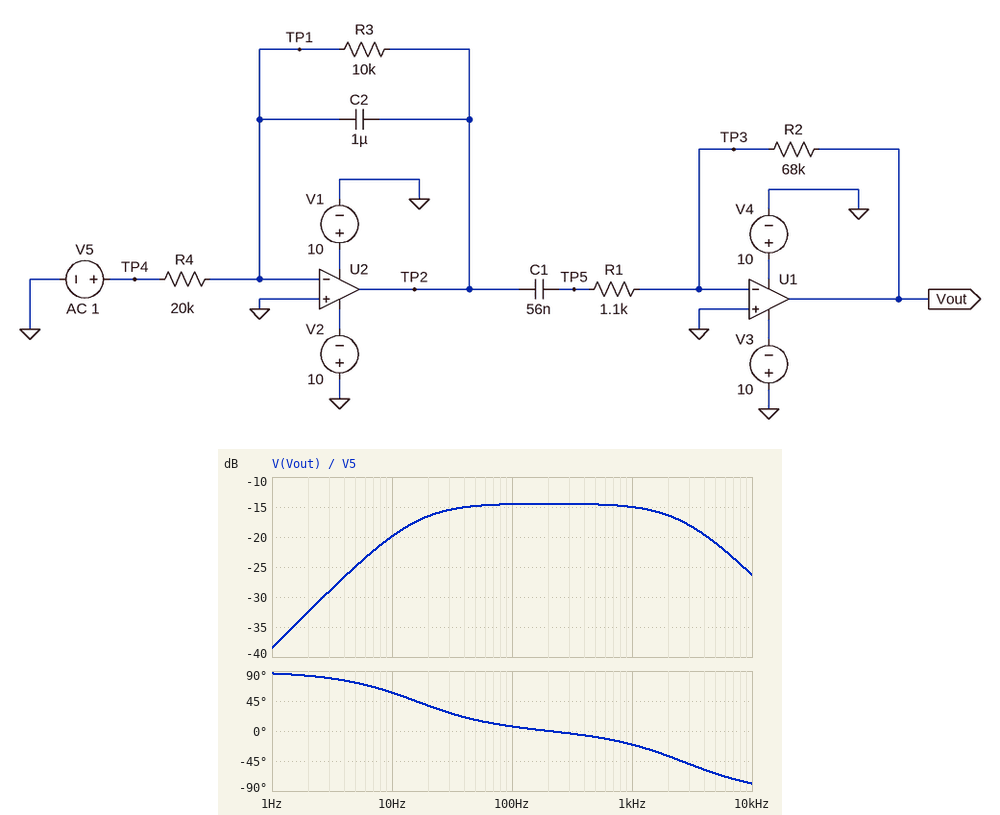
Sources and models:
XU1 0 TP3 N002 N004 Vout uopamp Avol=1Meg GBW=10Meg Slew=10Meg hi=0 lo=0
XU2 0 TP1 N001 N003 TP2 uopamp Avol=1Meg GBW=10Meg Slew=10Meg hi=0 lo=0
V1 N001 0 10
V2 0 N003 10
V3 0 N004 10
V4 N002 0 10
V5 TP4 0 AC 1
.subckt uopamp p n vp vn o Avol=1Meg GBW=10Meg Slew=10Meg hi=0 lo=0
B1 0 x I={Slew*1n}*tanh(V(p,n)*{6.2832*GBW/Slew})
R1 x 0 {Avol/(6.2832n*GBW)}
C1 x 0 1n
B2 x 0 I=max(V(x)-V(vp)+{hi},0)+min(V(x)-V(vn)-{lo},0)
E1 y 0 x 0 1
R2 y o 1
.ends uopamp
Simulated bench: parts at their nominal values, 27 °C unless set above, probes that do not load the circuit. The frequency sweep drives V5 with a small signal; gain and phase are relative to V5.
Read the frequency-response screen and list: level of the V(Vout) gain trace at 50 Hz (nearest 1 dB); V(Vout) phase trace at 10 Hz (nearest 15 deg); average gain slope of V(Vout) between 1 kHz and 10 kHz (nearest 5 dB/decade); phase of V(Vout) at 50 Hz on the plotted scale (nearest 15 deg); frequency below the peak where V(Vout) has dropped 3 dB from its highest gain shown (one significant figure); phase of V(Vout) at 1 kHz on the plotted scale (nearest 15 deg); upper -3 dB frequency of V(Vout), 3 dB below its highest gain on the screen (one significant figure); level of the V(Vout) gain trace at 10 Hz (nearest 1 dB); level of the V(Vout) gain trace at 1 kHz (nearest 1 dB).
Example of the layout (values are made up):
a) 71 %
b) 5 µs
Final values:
a) -15 dB
b) 60 deg
c) -10 dB/decade
d) 15 deg
e) 20 Hz
f) -15 deg
g) 3 kHz
h) -20 dB
i) -15 dB
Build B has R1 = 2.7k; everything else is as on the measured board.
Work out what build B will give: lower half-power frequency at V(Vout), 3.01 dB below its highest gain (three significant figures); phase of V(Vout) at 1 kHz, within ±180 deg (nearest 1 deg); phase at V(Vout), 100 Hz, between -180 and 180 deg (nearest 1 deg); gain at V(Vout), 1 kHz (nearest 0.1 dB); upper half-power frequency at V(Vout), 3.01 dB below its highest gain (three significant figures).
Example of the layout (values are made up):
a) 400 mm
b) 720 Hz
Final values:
a) 15.5 Hz
b) -43 deg
c) 4 deg
d) -17.2 dB
e) 1.09 kHz
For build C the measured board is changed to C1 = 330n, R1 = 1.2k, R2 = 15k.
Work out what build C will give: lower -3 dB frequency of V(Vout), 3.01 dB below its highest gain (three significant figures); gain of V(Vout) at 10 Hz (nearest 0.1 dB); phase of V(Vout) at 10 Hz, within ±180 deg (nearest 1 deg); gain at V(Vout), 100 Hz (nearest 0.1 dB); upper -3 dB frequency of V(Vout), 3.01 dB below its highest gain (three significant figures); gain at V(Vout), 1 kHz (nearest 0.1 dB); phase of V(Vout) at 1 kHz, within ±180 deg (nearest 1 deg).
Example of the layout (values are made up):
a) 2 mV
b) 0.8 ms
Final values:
a) 14.8 Hz
b) -17.6 dB
c) 56 deg
d) -12.5 dB
e) 433 Hz
f) -20.7 dB
g) -67 deg
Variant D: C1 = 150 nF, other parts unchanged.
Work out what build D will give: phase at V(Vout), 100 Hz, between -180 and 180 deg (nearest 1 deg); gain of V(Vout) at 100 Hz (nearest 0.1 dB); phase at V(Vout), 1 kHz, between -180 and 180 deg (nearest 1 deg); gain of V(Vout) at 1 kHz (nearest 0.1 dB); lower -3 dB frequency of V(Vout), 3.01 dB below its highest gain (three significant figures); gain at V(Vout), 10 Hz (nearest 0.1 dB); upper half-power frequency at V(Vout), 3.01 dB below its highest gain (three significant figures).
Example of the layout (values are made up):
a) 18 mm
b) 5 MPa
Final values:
a) 3 deg
b) -6.0 dB
c) -45 deg
d) -9.0 dB
e) 15.4 Hz
f) -11.3 dB
g) 1.00 kHz
